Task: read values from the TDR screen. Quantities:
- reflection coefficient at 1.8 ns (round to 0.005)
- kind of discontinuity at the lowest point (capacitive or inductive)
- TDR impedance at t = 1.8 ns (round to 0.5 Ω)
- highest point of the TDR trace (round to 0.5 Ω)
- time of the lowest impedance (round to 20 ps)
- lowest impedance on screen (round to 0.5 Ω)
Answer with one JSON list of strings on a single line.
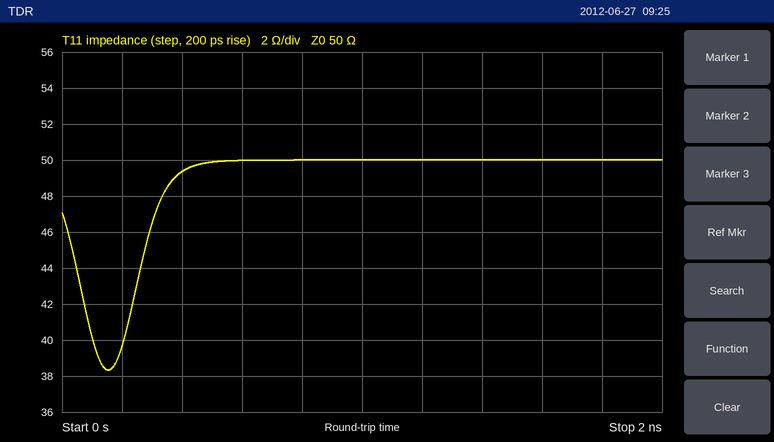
["0.000", "capacitive", "50.0 Ω", "50.0 Ω", "160 ps", "38.5 Ω"]
